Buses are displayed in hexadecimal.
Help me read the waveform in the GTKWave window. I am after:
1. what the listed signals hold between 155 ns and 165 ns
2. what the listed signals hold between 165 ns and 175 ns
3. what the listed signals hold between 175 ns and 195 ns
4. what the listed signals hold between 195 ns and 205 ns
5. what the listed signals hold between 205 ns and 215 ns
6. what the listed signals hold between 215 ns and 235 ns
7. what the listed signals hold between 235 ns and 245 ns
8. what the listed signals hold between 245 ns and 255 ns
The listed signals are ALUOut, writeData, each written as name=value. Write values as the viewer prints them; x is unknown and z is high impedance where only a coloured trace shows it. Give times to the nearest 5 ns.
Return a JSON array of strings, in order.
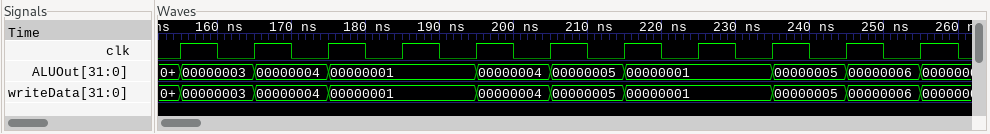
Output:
["ALUOut=00000003, writeData=00000003", "ALUOut=00000004, writeData=00000004", "ALUOut=00000001, writeData=00000001", "ALUOut=00000004, writeData=00000004", "ALUOut=00000005, writeData=00000005", "ALUOut=00000001, writeData=00000001", "ALUOut=00000005, writeData=00000005", "ALUOut=00000006, writeData=00000006"]
